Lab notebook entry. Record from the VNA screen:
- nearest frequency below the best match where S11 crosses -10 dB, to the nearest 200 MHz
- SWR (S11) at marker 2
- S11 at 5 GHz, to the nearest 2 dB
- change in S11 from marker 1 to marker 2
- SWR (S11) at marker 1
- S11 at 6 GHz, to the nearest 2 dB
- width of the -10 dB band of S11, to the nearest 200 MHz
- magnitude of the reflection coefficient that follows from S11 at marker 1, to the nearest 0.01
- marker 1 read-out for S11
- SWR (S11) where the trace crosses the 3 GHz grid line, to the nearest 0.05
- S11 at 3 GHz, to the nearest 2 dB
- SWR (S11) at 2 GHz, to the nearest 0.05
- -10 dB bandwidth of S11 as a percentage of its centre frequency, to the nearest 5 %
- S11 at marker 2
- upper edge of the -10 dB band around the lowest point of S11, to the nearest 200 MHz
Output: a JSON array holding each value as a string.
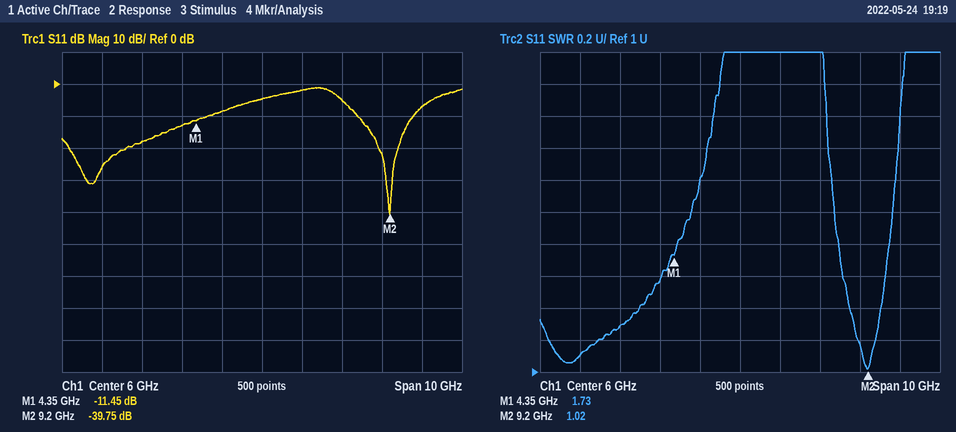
["8.4 GHz", "1.02", "-8 dB", "-28.30 dB", "1.73", "-4 dB", "1.4 GHz", "0.27", "-11.45 dB", "1.30", "-18 dB", "1.10", "15 %", "-39.75 dB", "9.8 GHz"]
